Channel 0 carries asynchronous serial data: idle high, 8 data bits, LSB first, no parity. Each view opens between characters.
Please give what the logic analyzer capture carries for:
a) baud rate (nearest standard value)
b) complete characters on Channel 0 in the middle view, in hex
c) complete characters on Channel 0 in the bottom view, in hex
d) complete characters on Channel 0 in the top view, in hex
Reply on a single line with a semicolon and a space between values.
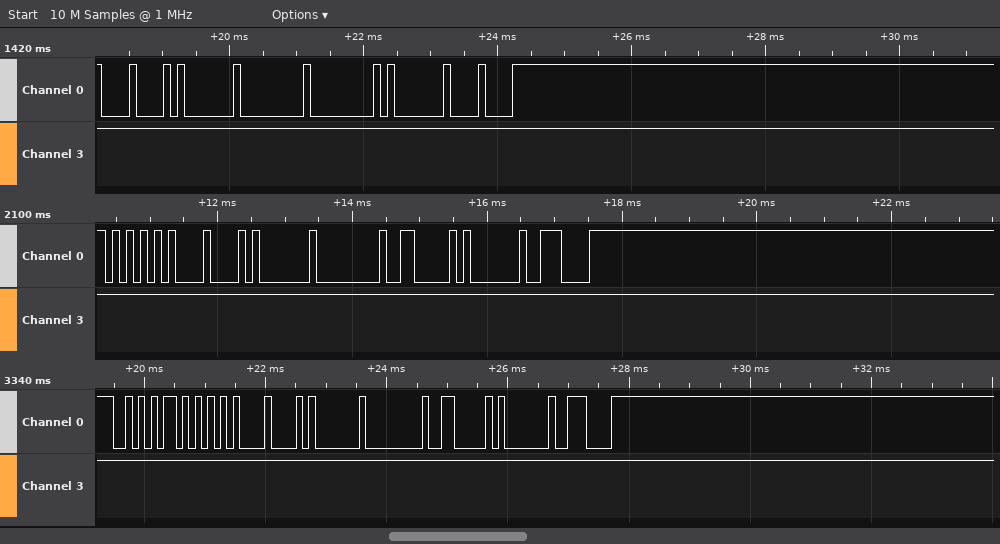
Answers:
9600 baud; 55, 08, 01, 00, 06, 01, 0E; AA, 55, 08, 01, 00, 06, 01, 0E; 08, 01, 00, 00, 01, 08
